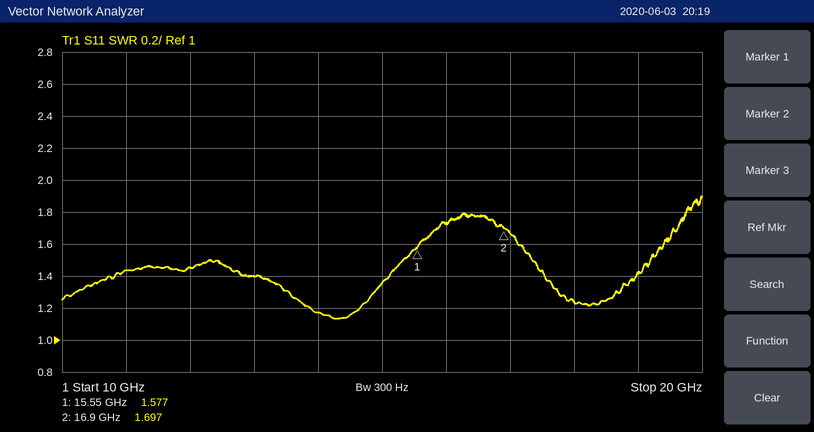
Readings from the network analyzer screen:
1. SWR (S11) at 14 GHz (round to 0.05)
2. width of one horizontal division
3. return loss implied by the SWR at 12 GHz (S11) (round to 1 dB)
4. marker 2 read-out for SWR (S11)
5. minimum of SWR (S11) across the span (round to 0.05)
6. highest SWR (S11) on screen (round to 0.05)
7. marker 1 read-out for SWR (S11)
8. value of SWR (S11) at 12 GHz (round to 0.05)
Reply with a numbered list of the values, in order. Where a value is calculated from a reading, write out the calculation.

1. 1.15
2. 1 GHz
3. −20 log10((1.45 − 1)/(1.45 + 1)) ≈ 15 dB
4. 1.697
5. 1.15
6. 1.90
7. 1.577
8. 1.45
